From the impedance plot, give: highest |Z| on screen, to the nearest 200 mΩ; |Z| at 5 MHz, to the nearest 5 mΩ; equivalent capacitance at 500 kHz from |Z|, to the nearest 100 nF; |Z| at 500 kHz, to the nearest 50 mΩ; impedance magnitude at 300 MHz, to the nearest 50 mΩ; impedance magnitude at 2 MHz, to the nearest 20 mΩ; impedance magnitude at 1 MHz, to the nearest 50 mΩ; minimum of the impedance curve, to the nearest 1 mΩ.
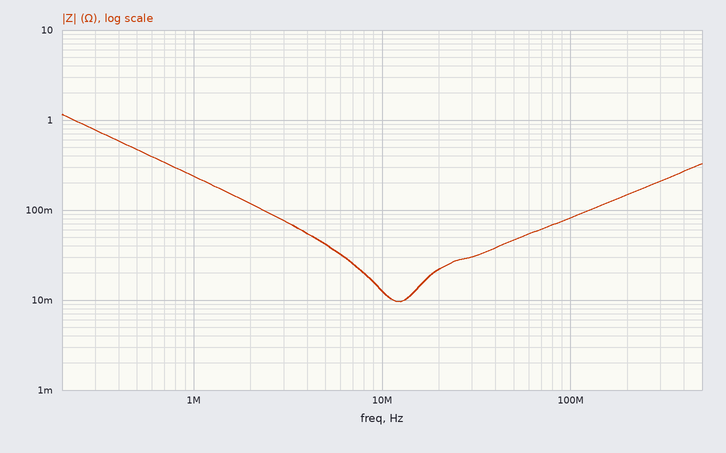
1.2 Ω
40 mΩ
700 nF
450 mΩ
200 mΩ
120 mΩ
250 mΩ
10 mΩ
